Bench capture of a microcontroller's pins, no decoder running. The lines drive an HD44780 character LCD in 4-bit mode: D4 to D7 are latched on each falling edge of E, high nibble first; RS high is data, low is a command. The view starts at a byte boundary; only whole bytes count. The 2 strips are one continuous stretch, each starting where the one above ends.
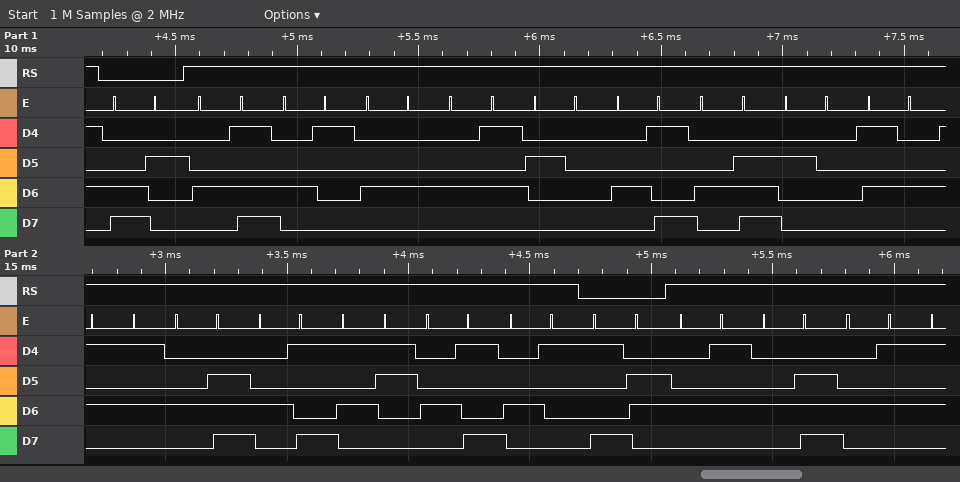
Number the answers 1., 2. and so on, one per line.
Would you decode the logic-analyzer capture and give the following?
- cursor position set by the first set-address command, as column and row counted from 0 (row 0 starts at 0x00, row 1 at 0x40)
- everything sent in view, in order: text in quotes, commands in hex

1. column 2, row 1
2. 0xC2 "MADE IN TUNISIA" 0x96 "ENE"
